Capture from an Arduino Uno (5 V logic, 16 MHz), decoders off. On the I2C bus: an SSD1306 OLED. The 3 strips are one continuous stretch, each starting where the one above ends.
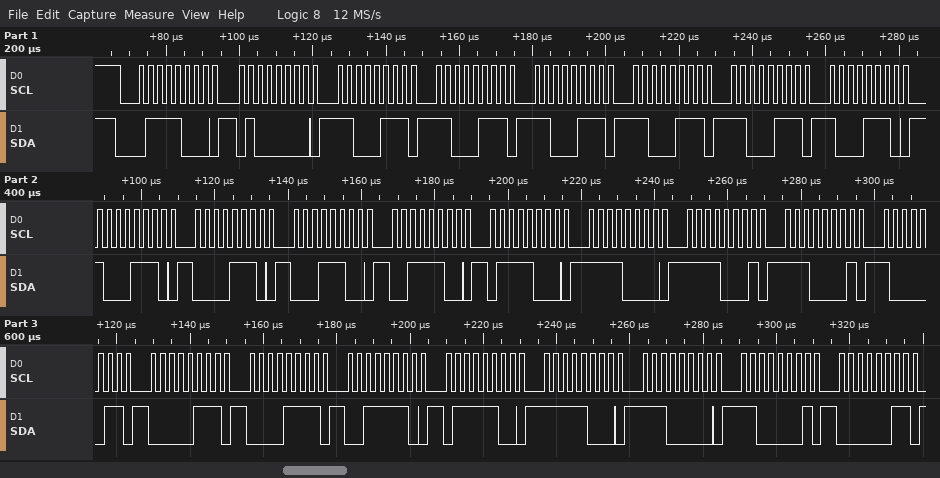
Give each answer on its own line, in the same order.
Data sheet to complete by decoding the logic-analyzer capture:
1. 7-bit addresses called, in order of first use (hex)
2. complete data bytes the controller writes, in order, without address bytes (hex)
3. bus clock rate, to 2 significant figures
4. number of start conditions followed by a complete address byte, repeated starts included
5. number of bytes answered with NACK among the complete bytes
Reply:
0x3C
40 C7 C7 C7 C7 C7 8E 8E 0E 1C 3C 78 F0 F1 E1 83 07 0F 3E 7C F8 E0 C1 03
400 kHz
1
0
